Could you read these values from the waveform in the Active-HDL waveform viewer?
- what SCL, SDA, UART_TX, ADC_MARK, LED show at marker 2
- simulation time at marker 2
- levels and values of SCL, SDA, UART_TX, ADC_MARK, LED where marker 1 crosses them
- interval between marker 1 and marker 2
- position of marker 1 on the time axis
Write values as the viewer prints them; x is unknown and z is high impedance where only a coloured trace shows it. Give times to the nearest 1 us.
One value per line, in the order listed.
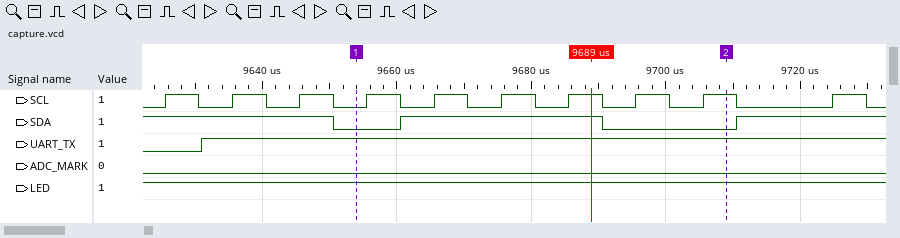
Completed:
SCL=1, SDA=0, UART_TX=1, ADC_MARK=0, LED=1
9709 us
SCL=0, SDA=0, UART_TX=1, ADC_MARK=0, LED=1
55 us
9654 us
